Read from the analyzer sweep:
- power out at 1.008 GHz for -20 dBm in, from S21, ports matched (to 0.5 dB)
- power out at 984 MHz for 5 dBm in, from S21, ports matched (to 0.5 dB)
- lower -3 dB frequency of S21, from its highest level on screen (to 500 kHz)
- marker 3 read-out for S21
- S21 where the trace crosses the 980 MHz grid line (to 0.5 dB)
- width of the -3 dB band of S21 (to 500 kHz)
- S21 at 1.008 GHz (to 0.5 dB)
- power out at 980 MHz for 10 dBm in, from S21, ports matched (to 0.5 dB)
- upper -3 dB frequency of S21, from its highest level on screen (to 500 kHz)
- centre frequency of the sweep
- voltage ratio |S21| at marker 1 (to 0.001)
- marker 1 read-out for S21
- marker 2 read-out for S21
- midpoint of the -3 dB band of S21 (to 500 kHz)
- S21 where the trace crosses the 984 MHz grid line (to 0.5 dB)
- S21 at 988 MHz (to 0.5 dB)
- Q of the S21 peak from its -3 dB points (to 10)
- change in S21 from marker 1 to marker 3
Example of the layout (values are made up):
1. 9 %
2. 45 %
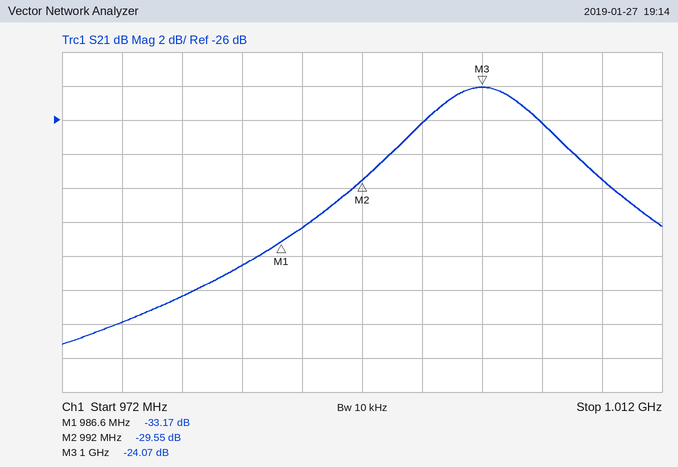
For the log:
1. -49.5 dBm
2. -29.5 dBm
3. 995.0 MHz
4. -24.07 dB
5. -36.5 dB
6. 10.0 MHz
7. -29.5 dB
8. -26.5 dBm
9. 1.0050 GHz
10. 992 MHz
11. 0.022
12. -33.17 dB
13. -29.55 dB
14. 1.0000 GHz
15. -34.5 dB
16. -32.5 dB
17. 100
18. 9.10 dB
